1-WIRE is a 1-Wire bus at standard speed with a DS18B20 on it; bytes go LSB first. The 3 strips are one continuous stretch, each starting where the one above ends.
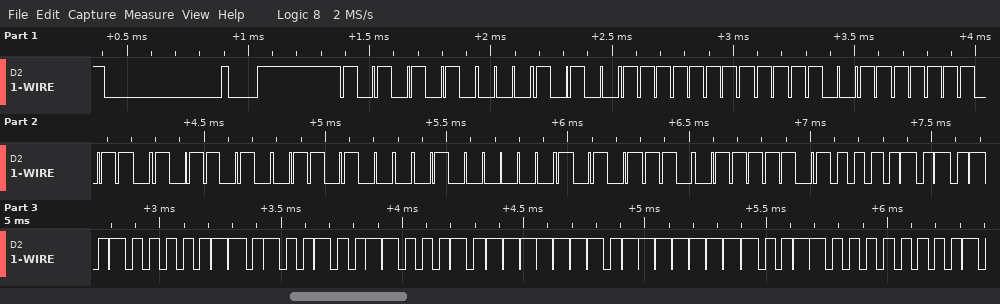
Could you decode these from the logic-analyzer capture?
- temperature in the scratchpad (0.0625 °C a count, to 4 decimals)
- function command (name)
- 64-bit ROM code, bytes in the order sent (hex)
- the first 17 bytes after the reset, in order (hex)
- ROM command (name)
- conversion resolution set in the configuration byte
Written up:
85.0000 °C
Read Scratchpad
28 FF CF DF 5A 16 02 75
55 28 FF CF DF 5A 16 02 75 BE 50 05 4B 46 7F FF 0C
Match ROM
12 bits
